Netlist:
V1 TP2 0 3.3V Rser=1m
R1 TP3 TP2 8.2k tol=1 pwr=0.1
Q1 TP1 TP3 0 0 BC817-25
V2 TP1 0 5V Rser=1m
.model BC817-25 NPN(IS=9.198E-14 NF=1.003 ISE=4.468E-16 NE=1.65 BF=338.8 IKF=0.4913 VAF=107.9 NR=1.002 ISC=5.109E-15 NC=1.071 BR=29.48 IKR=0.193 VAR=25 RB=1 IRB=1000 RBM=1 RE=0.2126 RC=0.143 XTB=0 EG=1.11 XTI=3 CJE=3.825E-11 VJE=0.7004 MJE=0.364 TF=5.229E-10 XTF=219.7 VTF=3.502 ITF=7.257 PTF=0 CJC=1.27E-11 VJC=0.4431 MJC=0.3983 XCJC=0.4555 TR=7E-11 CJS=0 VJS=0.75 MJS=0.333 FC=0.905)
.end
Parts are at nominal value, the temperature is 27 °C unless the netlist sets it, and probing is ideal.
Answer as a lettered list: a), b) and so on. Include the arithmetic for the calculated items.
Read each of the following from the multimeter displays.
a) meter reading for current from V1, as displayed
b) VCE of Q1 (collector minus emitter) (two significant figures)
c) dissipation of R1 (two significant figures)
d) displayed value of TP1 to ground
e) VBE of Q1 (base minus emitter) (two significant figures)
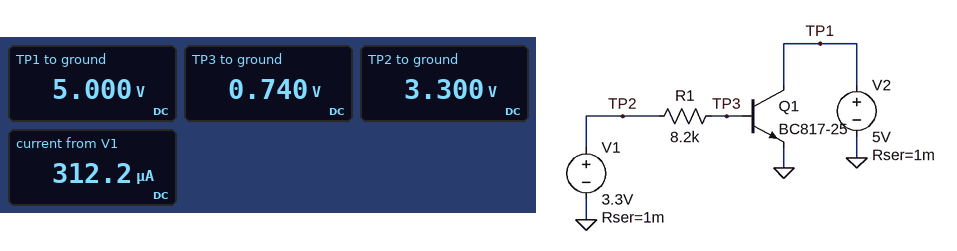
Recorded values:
a) 312.2 µA
b) 5 V = 5.0 V
c) (3.3 V - 740 mV)^2 / 8.2 kΩ = 800 µW
d) 5.000 V
e) 740 mV = 740 mV
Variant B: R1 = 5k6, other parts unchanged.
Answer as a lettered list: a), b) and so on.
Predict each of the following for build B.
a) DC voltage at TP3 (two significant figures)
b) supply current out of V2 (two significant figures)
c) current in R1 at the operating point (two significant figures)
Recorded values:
a) 760 mV
b) 120 mA
c) 450 µA
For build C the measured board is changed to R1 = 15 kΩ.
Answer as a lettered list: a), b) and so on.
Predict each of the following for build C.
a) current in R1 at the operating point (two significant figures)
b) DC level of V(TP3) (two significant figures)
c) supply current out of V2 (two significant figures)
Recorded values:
a) 170 µA
b) 720 mV
c) 53 mA
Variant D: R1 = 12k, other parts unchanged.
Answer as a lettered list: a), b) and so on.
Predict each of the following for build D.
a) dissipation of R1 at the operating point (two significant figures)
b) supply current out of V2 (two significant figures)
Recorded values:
a) 550 µW
b) 65 mA
